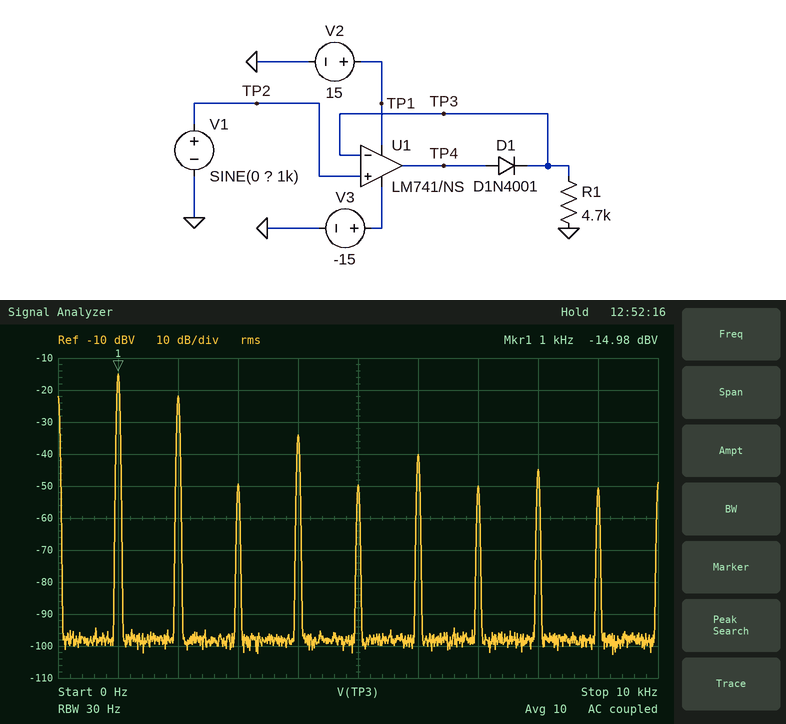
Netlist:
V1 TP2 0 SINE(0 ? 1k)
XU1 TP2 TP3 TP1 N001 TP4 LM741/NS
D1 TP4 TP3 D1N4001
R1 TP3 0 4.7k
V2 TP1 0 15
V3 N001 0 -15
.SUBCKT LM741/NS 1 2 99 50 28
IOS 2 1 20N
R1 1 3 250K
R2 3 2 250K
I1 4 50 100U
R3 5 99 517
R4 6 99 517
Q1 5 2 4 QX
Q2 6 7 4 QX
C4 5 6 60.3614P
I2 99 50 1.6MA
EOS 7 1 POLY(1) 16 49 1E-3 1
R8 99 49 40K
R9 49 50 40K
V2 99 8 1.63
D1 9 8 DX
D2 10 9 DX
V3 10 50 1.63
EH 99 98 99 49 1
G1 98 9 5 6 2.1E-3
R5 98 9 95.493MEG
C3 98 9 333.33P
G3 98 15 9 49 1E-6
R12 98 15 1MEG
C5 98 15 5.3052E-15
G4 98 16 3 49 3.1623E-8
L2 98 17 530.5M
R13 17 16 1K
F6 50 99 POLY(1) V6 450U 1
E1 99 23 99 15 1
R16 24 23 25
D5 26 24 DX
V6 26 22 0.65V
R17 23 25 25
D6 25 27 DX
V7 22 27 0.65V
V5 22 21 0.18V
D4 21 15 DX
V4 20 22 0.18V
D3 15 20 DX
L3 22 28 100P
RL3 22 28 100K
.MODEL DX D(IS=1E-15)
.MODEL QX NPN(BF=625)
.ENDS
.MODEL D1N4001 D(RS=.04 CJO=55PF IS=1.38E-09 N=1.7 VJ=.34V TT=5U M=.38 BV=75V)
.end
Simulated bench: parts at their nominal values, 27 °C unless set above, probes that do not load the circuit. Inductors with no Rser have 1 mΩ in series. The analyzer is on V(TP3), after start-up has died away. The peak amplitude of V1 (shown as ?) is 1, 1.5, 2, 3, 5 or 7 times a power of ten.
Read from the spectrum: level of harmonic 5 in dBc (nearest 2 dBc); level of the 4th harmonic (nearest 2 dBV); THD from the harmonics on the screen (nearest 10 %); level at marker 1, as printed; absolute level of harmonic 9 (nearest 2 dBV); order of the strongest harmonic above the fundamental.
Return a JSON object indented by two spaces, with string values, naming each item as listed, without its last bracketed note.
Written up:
{
  "level of harmonic 5 in dBc": "-34 dBc",
  "level of the 4th harmonic": "-34 dBV",
  "THD from the harmonics on the screen": "50 %",
  "level at marker 1, as printed": "-14.98 dBV",
  "absolute level of harmonic 9": "-50 dBV",
  "order of the strongest harmonic above the fundamental": "2"
}
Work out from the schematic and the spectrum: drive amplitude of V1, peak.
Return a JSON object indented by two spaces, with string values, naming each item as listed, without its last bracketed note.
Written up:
{
  "drive amplitude of V1, peak": "500 mV"
}
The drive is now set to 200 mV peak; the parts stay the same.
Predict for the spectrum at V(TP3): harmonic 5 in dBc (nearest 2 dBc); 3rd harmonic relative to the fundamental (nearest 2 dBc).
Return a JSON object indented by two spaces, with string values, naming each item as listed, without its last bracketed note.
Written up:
{
  "harmonic 5 in dBc": "-34 dBc",
  "3rd harmonic relative to the fundamental": "-32 dBc"
}
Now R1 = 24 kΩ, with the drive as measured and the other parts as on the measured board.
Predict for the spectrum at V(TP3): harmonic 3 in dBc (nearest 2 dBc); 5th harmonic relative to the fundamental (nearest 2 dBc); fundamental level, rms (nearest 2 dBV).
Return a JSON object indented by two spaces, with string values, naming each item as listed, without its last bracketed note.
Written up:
{
  "harmonic 3 in dBc": "-30 dBc",
  "5th harmonic relative to the fundamental": "-32 dBc",
  "fundamental level, rms": "-14 dBV"
}
